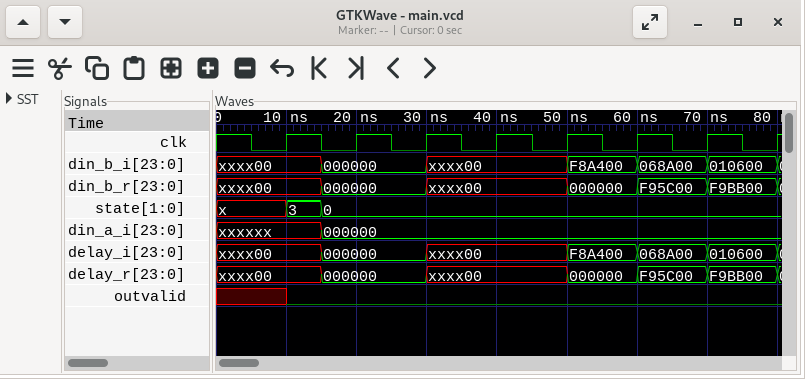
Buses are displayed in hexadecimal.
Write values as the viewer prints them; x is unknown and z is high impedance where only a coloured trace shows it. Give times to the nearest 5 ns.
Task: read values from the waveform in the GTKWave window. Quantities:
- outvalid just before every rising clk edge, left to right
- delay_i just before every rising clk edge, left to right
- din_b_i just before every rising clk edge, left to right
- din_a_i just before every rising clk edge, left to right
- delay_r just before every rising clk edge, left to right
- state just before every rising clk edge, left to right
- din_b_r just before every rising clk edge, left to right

x 0 0 0 0 0 0 0
xxxx00, 000000, 000000, xxxx00, xxxx00, F8A400, 068A00, 010600
xxxx00, 000000, 000000, xxxx00, xxxx00, F8A400, 068A00, 010600
xxxxxx, 000000, 000000, 000000, 000000, 000000, 000000, 000000
xxxx00, 000000, 000000, xxxx00, xxxx00, 000000, F95C00, F9BB00
x, 0, 0, 0, 0, 0, 0, 0
xxxx00, 000000, 000000, xxxx00, xxxx00, 000000, F95C00, F9BB00
